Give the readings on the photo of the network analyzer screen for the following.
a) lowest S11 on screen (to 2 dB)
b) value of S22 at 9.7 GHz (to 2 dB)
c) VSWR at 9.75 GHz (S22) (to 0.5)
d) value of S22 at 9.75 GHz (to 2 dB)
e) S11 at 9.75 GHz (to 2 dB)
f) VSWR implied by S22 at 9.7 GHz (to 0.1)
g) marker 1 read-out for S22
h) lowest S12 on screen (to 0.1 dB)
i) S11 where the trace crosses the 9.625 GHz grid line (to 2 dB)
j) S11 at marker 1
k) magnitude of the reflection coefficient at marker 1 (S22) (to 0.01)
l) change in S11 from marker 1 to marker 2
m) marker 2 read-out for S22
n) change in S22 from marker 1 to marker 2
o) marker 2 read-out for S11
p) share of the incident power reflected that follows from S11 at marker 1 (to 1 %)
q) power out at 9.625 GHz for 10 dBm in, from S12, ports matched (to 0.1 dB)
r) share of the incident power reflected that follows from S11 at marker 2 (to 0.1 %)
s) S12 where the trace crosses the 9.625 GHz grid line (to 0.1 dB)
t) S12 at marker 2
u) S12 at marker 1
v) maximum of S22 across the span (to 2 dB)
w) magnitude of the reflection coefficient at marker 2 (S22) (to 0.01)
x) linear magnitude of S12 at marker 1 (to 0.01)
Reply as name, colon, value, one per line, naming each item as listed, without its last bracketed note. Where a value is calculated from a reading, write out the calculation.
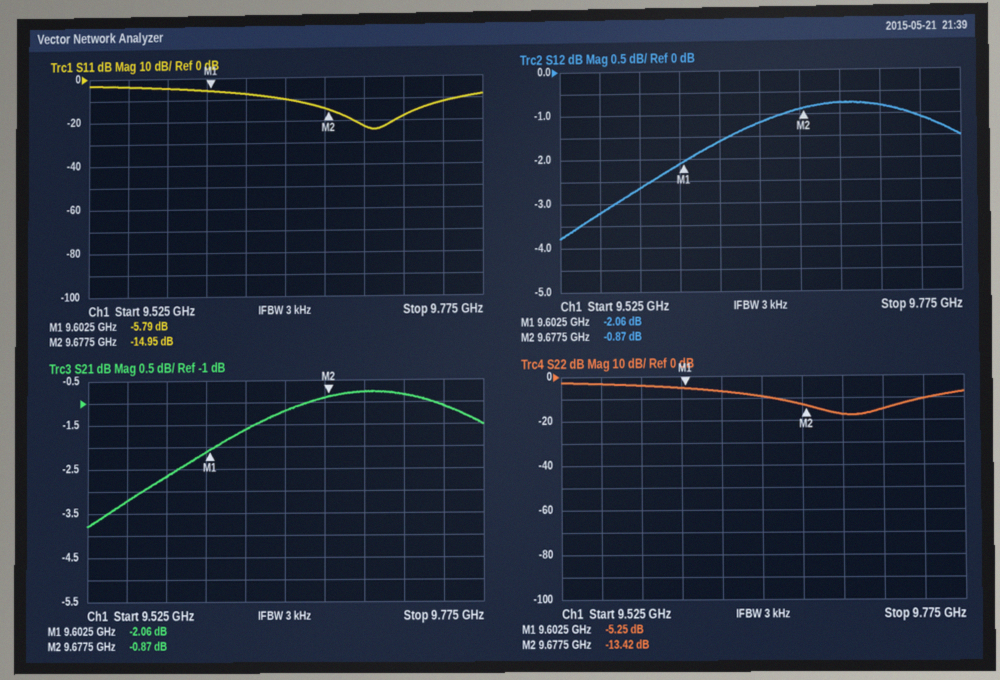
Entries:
lowest S11 on screen: -24 dB
value of S22 at 9.7 GHz: -18 dB
VSWR at 9.75 GHz (S22): |Γ| = 10^(-10/20) = 0.3162; VSWR = (1 + 0.3162)/(1 − 0.3162) ≈ 1.92, so 2.0 to the nearest 0.5
value of S22 at 9.75 GHz: -10 dB
S11 at 9.75 GHz: -12 dB
VSWR implied by S22 at 9.7 GHz: |Γ| = 10^(-18/20) = 0.1259; VSWR = (1 + 0.1259)/(1 − 0.1259) ≈ 1.3
marker 1 read-out for S22: -5.25 dB
lowest S12 on screen: -3.8 dB
S11 where the trace crosses the 9.625 GHz grid line: -8 dB
S11 at marker 1: -5.79 dB
magnitude of the reflection coefficient at marker 1 (S22): 10^(-5.25/20) ≈ 0.55
change in S11 from marker 1 to marker 2: -14.95 − (-5.79) = -9.16 dB
marker 2 read-out for S22: -13.42 dB
change in S22 from marker 1 to marker 2: -13.42 − (-5.25) = -8.17 dB
marker 2 read-out for S11: -14.95 dB
share of the incident power reflected that follows from S11 at marker 1: 10^(-5.79/10) ≈ 26 %
power out at 9.625 GHz for 10 dBm in, from S12, ports matched: 10 dBm + (-1.6 dB) = 8.4 dBm
share of the incident power reflected that follows from S11 at marker 2: 10^(-14.95/10) ≈ 3.2 %
S12 where the trace crosses the 9.625 GHz grid line: -1.6 dB
S12 at marker 2: -0.87 dB
S12 at marker 1: -2.06 dB
maximum of S22 across the span: -2 dB
magnitude of the reflection coefficient at marker 2 (S22): 10^(-13.42/20) ≈ 0.21
linear magnitude of S12 at marker 1: 10^(-2.06/20) ≈ 0.79
